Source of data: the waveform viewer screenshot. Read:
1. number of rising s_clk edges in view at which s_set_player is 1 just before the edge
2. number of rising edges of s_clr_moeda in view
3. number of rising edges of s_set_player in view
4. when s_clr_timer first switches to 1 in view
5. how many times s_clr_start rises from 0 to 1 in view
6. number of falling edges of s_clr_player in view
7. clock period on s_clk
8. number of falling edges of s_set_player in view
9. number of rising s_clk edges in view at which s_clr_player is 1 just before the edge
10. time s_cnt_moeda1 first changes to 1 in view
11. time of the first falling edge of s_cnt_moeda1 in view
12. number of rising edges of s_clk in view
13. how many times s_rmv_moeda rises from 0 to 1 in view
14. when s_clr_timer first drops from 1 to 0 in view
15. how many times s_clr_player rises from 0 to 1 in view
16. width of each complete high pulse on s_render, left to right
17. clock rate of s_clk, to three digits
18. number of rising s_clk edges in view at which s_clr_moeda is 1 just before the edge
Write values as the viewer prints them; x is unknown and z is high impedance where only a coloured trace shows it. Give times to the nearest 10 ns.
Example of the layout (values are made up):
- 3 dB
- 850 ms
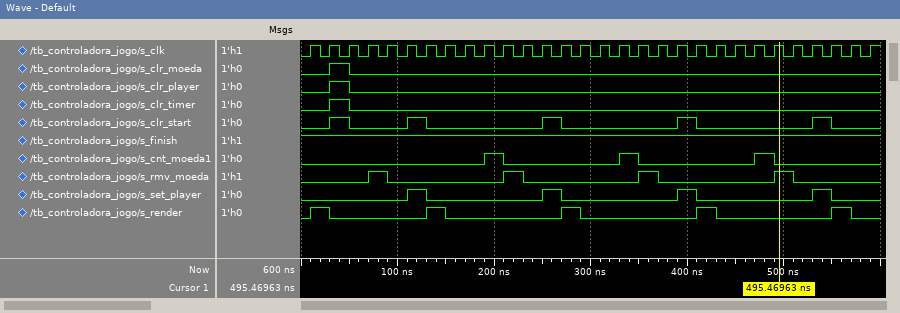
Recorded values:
- 4
- 1
- 4
- 30 ns
- 5
- 1
- 20 ns
- 4
- 1
- 190 ns
- 210 ns
- 30
- 4
- 50 ns
- 1
- 20 ns, 20 ns, 20 ns, 20 ns, 20 ns
- 50.0 MHz
- 1
